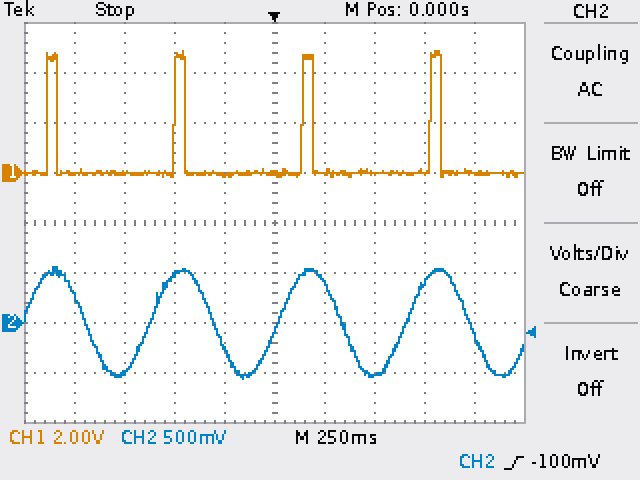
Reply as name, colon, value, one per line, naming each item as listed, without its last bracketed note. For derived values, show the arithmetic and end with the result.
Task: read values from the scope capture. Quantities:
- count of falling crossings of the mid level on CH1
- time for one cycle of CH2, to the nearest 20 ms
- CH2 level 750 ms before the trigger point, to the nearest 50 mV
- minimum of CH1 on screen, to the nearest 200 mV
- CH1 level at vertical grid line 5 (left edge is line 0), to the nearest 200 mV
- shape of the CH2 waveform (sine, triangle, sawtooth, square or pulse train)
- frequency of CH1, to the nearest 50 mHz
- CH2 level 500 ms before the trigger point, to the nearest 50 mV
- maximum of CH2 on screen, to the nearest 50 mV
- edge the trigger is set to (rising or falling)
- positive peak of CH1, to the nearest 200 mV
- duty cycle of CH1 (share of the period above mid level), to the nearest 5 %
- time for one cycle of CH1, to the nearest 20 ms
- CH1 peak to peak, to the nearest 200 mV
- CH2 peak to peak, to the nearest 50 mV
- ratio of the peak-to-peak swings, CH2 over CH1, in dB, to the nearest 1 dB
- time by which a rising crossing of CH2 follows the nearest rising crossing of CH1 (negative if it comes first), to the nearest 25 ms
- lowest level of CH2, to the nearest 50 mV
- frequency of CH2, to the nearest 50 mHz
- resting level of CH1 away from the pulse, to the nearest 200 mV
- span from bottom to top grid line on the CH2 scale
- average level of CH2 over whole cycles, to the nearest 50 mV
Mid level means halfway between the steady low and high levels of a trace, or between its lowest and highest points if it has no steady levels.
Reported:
count of falling crossings of the mid level on CH1: 4
time for one cycle of CH2, to the nearest 20 ms: 640 ms
CH2 level 750 ms before the trigger point, to the nearest 50 mV: -500 mV
minimum of CH1 on screen, to the nearest 200 mV: -200 mV
CH1 level at vertical grid line 5 (left edge is line 0), to the nearest 200 mV: 0.0 V
shape of the CH2 waveform: sine
frequency of CH1, to the nearest 50 mHz: 1 / 640 ms ≈ 1.56 Hz, so 1.55 Hz to the nearest 50 mHz
CH2 level 500 ms before the trigger point, to the nearest 50 mV: 450 mV
maximum of CH2 on screen, to the nearest 50 mV: 550 mV
edge the trigger is set to: rising
positive peak of CH1, to the nearest 200 mV: 4.8 V
duty cycle of CH1 (share of the period above mid level), to the nearest 5 %: 10 %
time for one cycle of CH1, to the nearest 20 ms: 640 ms
CH1 peak to peak, to the nearest 200 mV: 4.8 V − (-200 mV) = 5.0 V
CH2 peak to peak, to the nearest 50 mV: 550 mV − (-550 mV) = 1.10 V
ratio of the peak-to-peak swings, CH2 over CH1, in dB, to the nearest 1 dB: 20 log10(1.10 V / 5.0 V) ≈ -13 dB
time by which a rising crossing of CH2 follows the nearest rising crossing of CH1 (negative if it comes first), to the nearest 25 ms: -125 ms
lowest level of CH2, to the nearest 50 mV: -550 mV
frequency of CH2, to the nearest 50 mHz: 1 / 640 ms ≈ 1.56 Hz, so 1.55 Hz to the nearest 50 mHz
resting level of CH1 away from the pulse, to the nearest 200 mV: 0.0 V
span from bottom to top grid line on the CH2 scale: 4 V
average level of CH2 over whole cycles, to the nearest 50 mV: (550 mV + (-550 mV)) / 2 ≈ 0 mV
